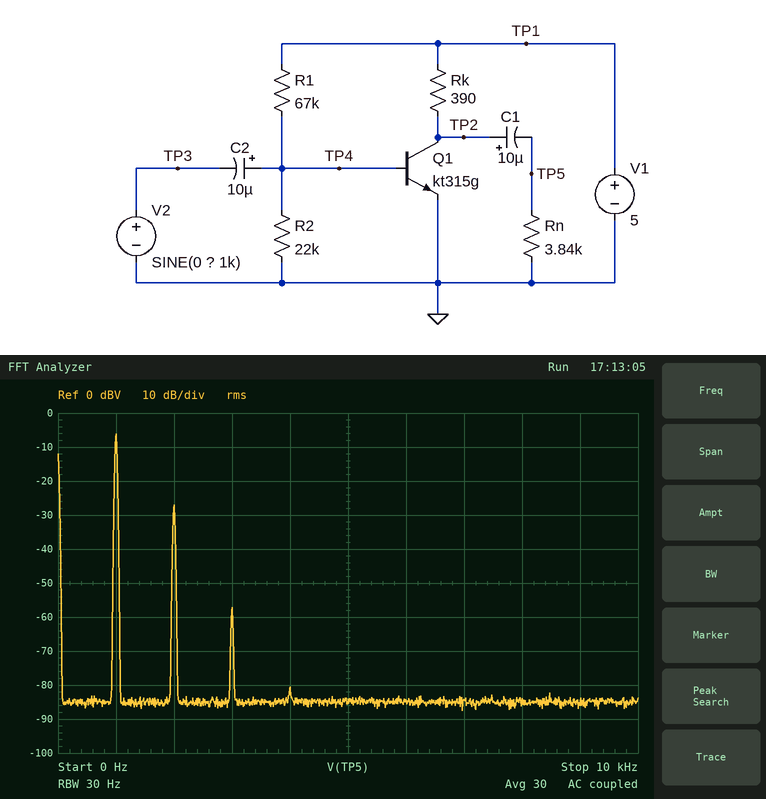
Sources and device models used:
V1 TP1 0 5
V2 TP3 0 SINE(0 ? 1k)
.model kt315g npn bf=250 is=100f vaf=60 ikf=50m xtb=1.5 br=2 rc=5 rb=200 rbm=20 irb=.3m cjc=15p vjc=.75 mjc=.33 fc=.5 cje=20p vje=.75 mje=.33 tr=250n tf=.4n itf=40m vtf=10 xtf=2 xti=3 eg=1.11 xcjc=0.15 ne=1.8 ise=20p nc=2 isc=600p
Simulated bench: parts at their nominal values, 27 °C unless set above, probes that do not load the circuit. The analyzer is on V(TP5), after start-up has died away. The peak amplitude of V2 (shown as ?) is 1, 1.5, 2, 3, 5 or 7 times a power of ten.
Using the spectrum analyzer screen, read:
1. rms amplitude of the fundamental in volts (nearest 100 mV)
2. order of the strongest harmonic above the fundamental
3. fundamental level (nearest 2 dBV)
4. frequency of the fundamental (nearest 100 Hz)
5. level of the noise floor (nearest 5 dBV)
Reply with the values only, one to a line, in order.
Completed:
500 mV
2
-6 dBV
1.0 kHz
-85 dBV
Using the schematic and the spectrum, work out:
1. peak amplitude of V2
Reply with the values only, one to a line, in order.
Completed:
15 mV
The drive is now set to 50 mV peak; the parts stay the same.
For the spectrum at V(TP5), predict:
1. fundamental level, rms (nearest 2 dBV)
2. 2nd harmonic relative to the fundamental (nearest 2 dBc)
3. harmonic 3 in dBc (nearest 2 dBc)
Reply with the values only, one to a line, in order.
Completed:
2 dBV
-10 dBc
-28 dBc
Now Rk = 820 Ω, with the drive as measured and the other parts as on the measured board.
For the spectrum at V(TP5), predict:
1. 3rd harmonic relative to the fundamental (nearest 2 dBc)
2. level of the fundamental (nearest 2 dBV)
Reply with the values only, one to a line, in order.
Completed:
-38 dBc
-2 dBV
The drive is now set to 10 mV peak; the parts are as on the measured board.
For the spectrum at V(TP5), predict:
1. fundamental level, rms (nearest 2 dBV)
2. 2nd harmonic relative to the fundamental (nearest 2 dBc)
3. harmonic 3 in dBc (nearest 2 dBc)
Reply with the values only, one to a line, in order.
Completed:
-10 dBV
-24 dBc
-58 dBc
